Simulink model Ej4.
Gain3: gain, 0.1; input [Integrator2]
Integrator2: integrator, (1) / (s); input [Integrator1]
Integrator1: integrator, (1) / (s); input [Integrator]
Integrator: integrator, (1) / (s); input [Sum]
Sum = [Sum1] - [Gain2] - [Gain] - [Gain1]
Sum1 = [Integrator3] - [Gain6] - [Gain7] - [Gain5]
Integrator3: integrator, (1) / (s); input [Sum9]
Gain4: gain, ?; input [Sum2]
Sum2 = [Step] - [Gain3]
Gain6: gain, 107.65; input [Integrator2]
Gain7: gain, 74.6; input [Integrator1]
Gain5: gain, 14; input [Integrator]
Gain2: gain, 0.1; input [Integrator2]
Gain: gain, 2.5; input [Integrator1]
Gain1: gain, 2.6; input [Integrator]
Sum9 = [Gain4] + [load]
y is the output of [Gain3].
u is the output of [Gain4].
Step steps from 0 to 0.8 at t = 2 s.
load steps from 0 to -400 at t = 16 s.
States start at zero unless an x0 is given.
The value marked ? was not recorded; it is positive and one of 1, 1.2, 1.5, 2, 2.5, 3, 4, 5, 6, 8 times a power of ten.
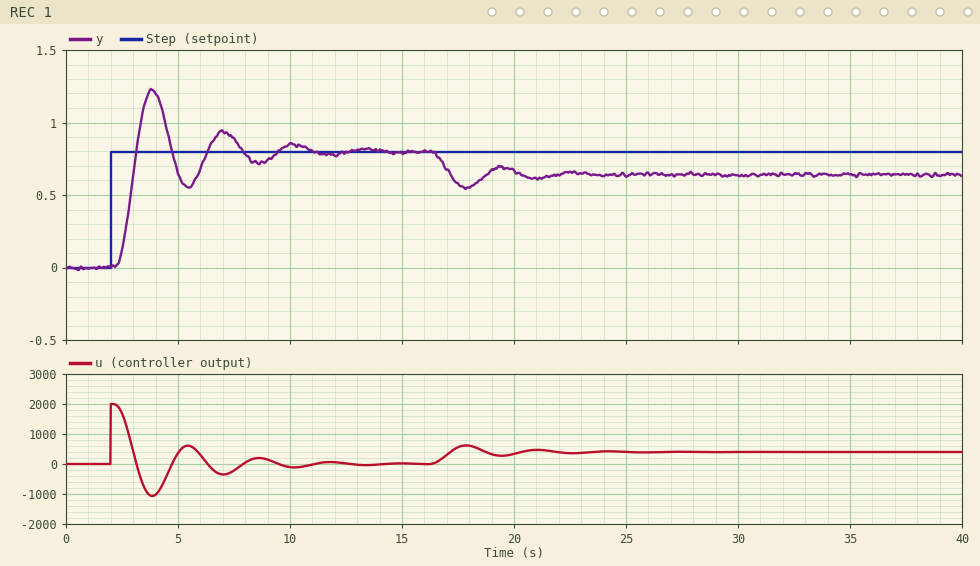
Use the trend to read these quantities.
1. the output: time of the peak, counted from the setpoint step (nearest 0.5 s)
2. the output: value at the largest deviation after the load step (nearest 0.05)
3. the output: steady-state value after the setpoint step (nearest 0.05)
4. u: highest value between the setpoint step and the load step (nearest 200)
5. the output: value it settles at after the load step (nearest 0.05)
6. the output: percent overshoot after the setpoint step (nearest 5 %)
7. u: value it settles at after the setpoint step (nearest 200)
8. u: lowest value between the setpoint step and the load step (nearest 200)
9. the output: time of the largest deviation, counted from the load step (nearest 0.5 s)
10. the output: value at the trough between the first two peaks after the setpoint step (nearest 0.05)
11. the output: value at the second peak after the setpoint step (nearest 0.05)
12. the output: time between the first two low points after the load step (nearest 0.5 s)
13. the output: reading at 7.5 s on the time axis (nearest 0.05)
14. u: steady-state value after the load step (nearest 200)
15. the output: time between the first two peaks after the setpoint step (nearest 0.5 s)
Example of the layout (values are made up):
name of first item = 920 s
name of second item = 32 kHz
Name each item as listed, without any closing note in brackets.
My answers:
the output: time of the peak, counted from the setpoint step = 2.0 s
the output: value at the largest deviation after the load step = 0.55
the output: steady-state value after the setpoint step = 0.80
u: highest value between the setpoint step and the load step = 2000
the output: value it settles at after the load step = 0.65
the output: percent overshoot after the setpoint step = 55 %
u: value it settles at after the setpoint step = 0
u: lowest value between the setpoint step and the load step = -1000
the output: time of the largest deviation, counted from the load step = 2.0 s
the output: value at the trough between the first two peaks after the setpoint step = 0.55
the output: value at the second peak after the setpoint step = 0.95
the output: time between the first two low points after the load step = 3.0 s
the output: reading at 7.5 s on the time axis = 0.90
u: steady-state value after the load step = 400
the output: time between the first two peaks after the setpoint step = 3.0 s
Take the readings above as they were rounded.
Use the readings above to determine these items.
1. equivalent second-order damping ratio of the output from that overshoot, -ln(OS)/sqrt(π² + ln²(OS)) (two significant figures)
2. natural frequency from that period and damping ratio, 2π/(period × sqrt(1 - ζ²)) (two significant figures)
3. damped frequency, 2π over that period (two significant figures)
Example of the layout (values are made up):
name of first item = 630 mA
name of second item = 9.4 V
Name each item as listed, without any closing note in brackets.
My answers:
equivalent second-order damping ratio of the output from that overshoot, -ln(OS)/sqrt(π² + ln²(OS)) = 0.19
natural frequency from that period and damping ratio, 2π/(period × sqrt(1 - ζ²)) = 2.1 rad/s
damped frequency, 2π over that period = 2.1 rad/s
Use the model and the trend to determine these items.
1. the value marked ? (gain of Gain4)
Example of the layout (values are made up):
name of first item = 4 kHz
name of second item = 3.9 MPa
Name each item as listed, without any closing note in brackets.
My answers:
the value marked ? = 2500
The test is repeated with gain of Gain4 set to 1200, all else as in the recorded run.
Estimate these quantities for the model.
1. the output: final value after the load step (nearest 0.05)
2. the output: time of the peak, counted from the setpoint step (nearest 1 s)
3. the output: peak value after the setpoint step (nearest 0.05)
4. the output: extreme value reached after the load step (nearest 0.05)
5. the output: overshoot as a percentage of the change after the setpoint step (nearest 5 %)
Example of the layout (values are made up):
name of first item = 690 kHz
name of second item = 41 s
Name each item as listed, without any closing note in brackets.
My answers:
the output: final value after the load step = 0.45
the output: time of the peak, counted from the setpoint step = 3 s
the output: peak value after the setpoint step = 0.95
the output: extreme value reached after the load step = 0.40
the output: overshoot as a percentage of the change after the setpoint step = 20 %
